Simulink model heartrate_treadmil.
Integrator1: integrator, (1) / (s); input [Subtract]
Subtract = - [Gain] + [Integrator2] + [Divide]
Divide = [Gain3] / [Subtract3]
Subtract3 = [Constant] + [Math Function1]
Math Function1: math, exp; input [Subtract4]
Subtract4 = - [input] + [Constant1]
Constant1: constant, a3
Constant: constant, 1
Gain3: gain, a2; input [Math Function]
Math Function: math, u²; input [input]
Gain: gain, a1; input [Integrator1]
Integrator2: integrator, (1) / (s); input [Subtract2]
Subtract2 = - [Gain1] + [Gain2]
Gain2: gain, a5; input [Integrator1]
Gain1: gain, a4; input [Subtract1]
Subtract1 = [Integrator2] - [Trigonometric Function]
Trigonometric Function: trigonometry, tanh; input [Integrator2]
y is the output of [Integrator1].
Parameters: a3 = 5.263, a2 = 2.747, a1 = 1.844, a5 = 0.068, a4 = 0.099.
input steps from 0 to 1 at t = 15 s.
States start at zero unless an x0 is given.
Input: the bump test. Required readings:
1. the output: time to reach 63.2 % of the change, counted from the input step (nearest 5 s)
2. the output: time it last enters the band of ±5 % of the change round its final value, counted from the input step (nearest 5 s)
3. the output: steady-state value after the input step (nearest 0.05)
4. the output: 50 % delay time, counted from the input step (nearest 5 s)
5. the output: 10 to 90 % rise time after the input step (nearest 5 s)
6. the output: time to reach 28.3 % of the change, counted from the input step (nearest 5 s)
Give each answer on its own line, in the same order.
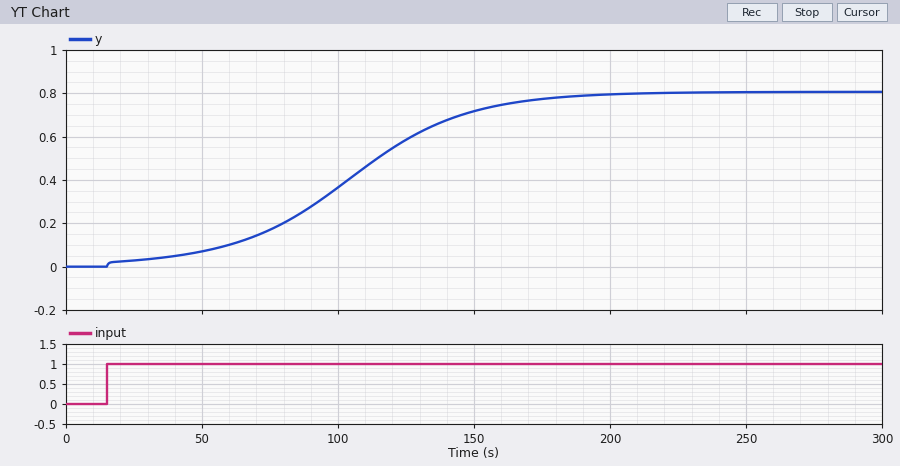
100 s
155 s
0.80
90 s
100 s
70 s
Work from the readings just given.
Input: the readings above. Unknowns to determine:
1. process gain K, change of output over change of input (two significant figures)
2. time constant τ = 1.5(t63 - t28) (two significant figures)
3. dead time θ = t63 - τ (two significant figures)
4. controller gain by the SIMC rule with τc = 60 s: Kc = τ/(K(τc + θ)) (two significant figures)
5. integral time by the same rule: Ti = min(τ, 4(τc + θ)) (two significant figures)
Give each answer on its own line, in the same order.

0.80
45 s
55 s
0.49
45 s
